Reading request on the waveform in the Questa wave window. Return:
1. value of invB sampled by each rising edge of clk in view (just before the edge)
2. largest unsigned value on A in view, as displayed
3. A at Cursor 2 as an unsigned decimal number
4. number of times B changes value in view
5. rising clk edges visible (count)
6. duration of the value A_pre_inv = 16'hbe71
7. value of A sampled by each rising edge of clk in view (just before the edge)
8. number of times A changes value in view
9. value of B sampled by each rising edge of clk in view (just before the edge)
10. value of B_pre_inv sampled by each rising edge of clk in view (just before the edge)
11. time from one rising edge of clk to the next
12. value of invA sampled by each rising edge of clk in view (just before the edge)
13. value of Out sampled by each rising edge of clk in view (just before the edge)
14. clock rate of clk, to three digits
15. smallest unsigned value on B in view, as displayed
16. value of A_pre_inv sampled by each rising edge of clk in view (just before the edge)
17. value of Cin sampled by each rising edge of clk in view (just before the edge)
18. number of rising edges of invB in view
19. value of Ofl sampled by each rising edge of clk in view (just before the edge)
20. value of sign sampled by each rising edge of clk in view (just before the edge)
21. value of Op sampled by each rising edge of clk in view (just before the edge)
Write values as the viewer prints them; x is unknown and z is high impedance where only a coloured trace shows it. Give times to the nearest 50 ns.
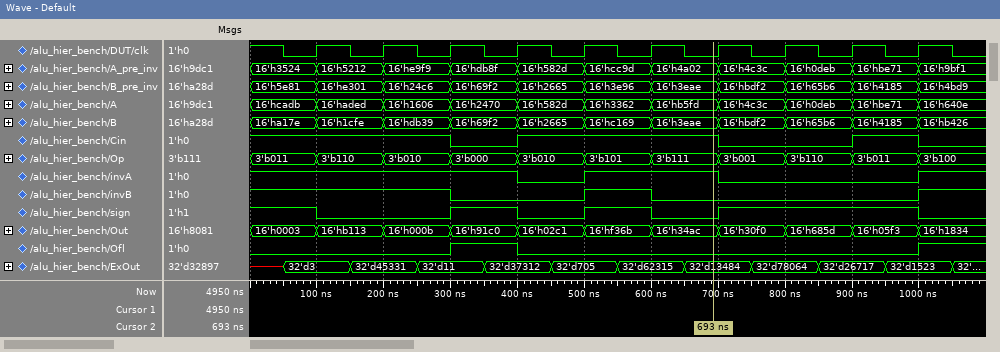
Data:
1 1 1 0 0 1 0 0 0 0
16'hcadb
46589
10
10
100 ns
16'hcadb, 16'haded, 16'h1606, 16'h2470, 16'h582d, 16'h3362, 16'hb5fd, 16'h4c3c, 16'h0deb, 16'hbe71
10
16'ha17e, 16'h1cfe, 16'hdb39, 16'h69f2, 16'h2665, 16'hc169, 16'h3eae, 16'hbdf2, 16'h65b6, 16'h4185
16'h5e81, 16'he301, 16'h24c6, 16'h69f2, 16'h2665, 16'h3e96, 16'h3eae, 16'hbdf2, 16'h65b6, 16'h4185
100 ns
1 1 1 1 0 1 1 0 0 0
16'h0003, 16'hb113, 16'h000b, 16'h91c0, 16'h02c1, 16'hf36b, 16'h34ac, 16'h30f0, 16'h685d, 16'h05f3
10.0 MHz
16'h1cfe
16'h3524, 16'h5212, 16'he9f9, 16'hdb8f, 16'h582d, 16'hcc9d, 16'h4a02, 16'h4c3c, 16'h0deb, 16'hbe71
1 1 1 0 1 1 1 0 0 1
2
0 0 0 1 0 0 0 0 0 0
1 0 0 1 0 1 0 1 1 1
3'b011, 3'b110, 3'b010, 3'b000, 3'b010, 3'b101, 3'b111, 3'b001, 3'b110, 3'b011
